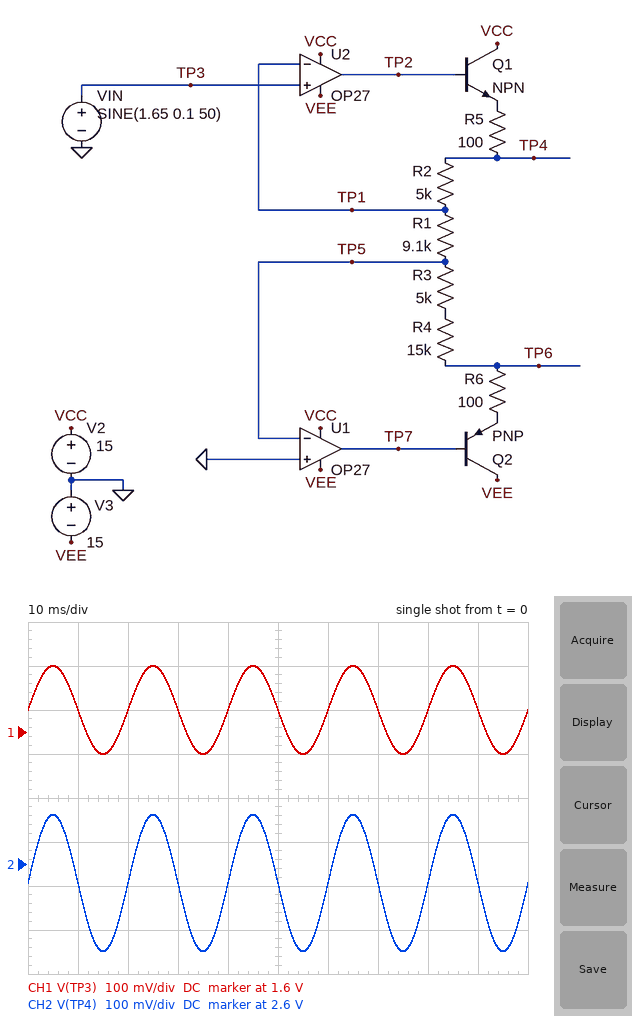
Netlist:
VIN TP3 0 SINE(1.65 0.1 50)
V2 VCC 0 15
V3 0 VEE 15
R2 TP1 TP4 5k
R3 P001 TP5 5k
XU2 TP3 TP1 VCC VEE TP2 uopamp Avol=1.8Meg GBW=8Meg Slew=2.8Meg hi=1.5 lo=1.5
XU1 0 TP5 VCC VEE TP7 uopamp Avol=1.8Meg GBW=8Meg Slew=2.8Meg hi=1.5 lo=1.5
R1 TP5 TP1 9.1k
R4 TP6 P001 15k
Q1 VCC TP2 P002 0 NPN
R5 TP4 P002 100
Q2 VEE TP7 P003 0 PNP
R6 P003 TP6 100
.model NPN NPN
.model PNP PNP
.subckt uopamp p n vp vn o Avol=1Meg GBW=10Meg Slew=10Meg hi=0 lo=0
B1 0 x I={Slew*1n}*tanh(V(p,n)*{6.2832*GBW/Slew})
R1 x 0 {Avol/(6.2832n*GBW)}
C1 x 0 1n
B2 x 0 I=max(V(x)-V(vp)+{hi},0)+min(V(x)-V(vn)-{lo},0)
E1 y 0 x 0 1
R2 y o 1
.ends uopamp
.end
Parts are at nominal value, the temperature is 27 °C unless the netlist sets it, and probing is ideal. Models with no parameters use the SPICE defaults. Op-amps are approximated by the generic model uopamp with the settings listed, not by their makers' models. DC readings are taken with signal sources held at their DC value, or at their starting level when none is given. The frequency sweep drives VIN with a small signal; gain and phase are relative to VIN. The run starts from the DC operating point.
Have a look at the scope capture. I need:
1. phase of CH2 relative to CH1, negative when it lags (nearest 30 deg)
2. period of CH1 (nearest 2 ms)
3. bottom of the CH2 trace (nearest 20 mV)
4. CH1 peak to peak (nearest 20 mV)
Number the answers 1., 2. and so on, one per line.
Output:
1. 0 deg
2. 20 ms
3. 2.40 V
4. 200 mV
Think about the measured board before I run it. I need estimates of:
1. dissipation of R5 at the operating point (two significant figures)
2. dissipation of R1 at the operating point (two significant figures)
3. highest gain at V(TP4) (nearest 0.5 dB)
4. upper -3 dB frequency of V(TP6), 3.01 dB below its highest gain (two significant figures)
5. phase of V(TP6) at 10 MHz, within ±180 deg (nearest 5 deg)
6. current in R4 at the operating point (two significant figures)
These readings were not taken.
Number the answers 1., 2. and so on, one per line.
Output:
1. 3.3 µW
2. 300 µW
3. 4.0 dB
4. 2.0 MHz
5. 50 deg
6. 180 µA
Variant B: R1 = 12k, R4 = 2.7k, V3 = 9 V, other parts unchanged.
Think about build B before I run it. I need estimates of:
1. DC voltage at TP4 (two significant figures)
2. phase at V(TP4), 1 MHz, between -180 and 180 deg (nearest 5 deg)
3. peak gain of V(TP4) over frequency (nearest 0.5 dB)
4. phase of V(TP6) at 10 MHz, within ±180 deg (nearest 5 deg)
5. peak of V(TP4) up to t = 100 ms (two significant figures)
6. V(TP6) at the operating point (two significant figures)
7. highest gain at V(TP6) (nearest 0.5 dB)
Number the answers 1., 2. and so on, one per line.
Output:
1. 2.3 V
2. -10 deg
3. 3.0 dB
4. 55 deg
5. 2.5 V
6. -1.1 V
7. -4.0 dB
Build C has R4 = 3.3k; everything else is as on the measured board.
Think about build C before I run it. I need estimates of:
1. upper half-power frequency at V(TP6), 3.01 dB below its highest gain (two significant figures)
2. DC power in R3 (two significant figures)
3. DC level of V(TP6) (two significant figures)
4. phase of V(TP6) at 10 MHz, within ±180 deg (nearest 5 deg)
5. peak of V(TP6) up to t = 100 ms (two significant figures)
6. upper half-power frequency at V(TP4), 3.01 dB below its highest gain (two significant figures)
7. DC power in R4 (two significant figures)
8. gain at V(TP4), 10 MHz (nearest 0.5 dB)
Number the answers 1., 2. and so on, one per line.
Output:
1. 2.8 MHz
2. 160 µW
3. -1.5 V
4. 55 deg
5. -1.4 V
6. 4.1 MHz
7. 110 µW
8. -3.5 dB
